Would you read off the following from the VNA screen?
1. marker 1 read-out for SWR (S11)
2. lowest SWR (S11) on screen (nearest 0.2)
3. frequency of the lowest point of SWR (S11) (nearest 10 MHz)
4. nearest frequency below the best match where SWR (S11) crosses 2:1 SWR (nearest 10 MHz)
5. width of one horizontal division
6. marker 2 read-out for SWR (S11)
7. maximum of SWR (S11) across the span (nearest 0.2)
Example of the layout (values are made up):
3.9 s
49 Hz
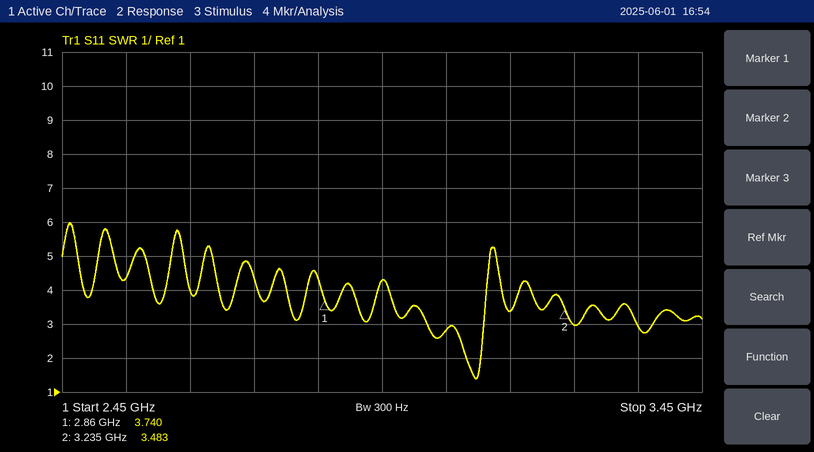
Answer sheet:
3.740
1.4
3.10 GHz
3.08 GHz
100 MHz
3.483
6.0
